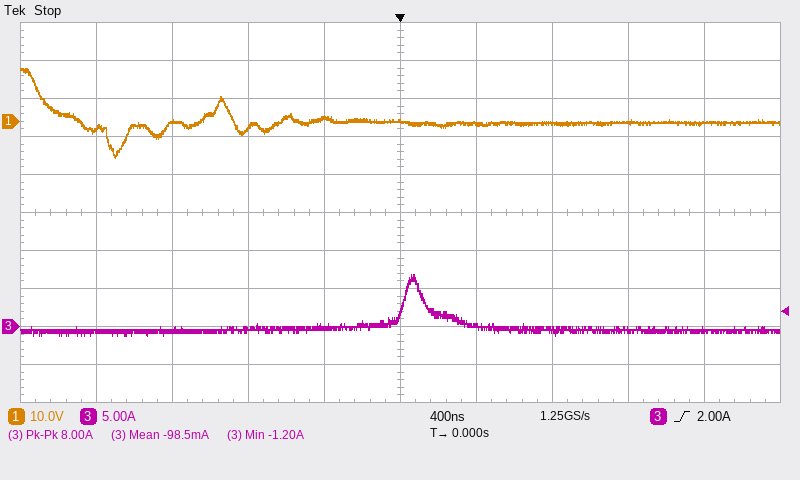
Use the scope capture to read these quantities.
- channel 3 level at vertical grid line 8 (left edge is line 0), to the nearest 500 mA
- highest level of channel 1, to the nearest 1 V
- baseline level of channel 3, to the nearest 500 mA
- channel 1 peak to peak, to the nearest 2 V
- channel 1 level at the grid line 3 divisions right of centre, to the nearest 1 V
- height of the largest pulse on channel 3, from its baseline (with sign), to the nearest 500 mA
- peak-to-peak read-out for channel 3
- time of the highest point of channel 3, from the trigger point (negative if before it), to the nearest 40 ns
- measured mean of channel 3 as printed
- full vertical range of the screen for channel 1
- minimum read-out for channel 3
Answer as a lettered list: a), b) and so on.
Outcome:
a) -500 mA
b) 14 V
c) -500 mA
d) 24 V
e) 0 V
f) +7.5 A
g) 8.00 A
h) +80 ns
i) -98.5 mA
j) 100 V
k) -1.20 A
